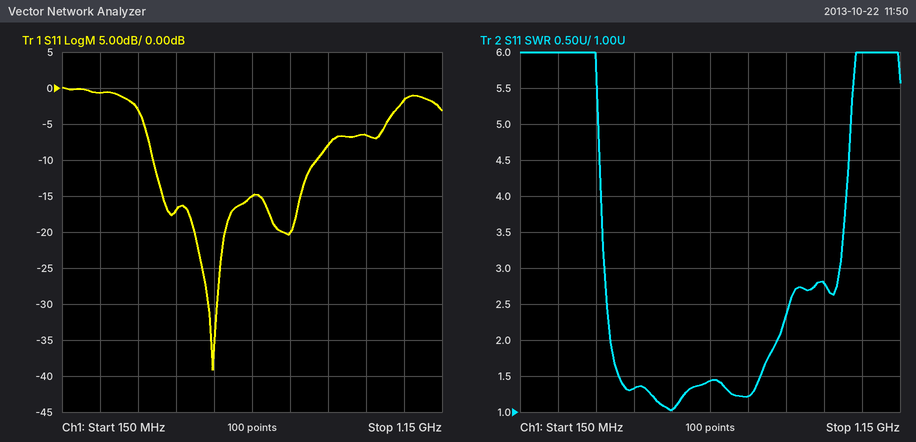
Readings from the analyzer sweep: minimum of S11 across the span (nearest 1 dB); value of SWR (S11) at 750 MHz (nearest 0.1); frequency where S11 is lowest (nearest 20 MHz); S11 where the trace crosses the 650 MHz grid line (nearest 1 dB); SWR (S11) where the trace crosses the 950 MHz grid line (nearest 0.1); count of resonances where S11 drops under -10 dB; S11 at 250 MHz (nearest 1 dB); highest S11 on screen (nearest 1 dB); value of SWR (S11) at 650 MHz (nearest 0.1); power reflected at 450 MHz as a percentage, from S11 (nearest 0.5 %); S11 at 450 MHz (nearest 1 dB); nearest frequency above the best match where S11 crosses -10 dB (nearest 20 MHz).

-39 dB
1.2
540 MHz
-15 dB
2.8
2
-1 dB
0 dB
1.4
2.0 %
-17 dB
820 MHz
